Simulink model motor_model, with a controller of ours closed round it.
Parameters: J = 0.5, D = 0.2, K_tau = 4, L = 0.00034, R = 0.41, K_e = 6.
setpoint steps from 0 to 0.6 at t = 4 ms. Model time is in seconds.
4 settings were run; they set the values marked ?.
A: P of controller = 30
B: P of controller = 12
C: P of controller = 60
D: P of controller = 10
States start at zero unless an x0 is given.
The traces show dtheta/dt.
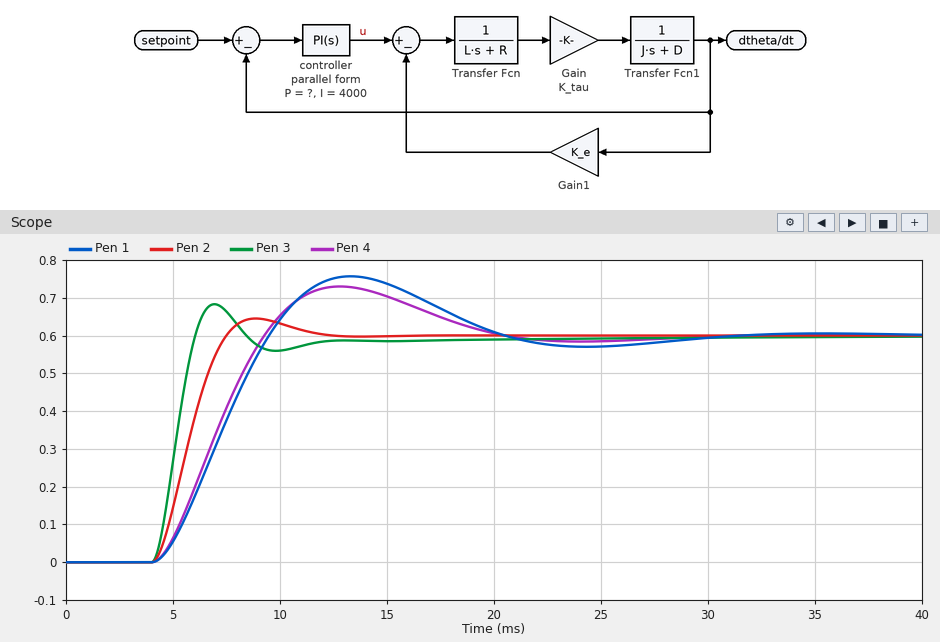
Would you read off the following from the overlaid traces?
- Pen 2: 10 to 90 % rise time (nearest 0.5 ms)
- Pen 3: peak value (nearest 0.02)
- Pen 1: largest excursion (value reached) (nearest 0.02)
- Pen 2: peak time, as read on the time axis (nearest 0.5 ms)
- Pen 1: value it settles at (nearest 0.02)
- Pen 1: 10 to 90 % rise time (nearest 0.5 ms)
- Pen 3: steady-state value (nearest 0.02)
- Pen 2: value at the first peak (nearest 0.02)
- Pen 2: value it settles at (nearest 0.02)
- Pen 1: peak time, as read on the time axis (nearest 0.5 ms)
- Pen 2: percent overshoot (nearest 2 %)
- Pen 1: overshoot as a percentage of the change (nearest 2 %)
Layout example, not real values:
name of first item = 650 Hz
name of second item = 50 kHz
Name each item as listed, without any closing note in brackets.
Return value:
Pen 2: 10 to 90 % rise time = 2.5 ms
Pen 3: peak value = 0.68
Pen 1: largest excursion (value reached) = 0.76
Pen 2: peak time, as read on the time axis = 9.0 ms
Pen 1: value it settles at = 0.60
Pen 1: 10 to 90 % rise time = 4.0 ms
Pen 3: steady-state value = 0.60
Pen 2: value at the first peak = 0.64
Pen 2: value it settles at = 0.60
Pen 1: peak time, as read on the time axis = 13.5 ms
Pen 2: percent overshoot = 8 %
Pen 1: overshoot as a percentage of the change = 26 %
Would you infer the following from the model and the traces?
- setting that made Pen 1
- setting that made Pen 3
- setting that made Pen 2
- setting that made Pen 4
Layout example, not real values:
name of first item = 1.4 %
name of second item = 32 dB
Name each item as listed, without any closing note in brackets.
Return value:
setting that made Pen 1 = D
setting that made Pen 3 = C
setting that made Pen 2 = A
setting that made Pen 4 = B
